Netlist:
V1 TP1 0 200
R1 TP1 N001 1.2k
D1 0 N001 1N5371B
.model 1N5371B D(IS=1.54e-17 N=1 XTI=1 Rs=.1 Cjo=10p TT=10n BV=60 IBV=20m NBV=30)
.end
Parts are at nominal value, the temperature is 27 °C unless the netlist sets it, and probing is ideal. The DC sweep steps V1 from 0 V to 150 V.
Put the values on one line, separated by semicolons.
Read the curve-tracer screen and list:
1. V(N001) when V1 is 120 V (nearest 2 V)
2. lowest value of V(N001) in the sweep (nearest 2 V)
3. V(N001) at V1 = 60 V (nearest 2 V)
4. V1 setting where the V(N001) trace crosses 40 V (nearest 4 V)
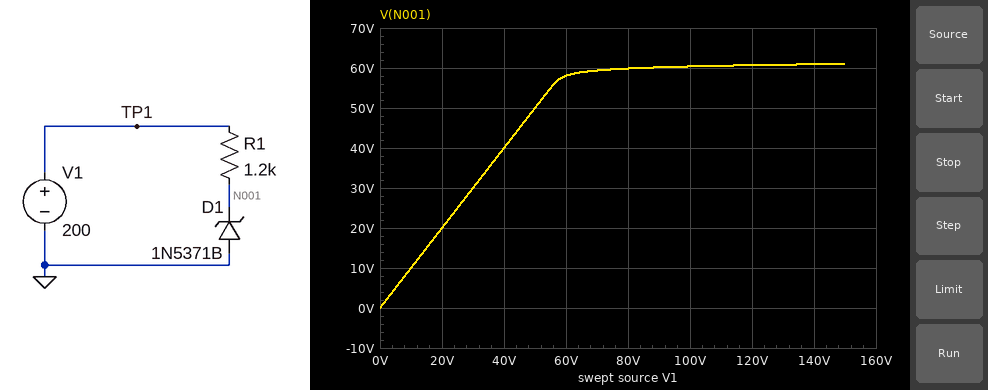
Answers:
60 V; 0 V; 58 V; 40 V
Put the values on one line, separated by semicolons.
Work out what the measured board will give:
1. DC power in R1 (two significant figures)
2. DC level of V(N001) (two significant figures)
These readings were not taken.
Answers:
16 W; 61 V
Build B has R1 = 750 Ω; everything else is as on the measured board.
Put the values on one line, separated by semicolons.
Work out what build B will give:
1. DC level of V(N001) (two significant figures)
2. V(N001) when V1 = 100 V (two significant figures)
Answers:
62 V; 61 V
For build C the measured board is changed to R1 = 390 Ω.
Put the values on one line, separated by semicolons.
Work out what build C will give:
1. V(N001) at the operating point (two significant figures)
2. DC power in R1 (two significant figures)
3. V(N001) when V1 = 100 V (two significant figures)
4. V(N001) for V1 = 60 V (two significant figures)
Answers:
62 V; 49 W; 61 V; 59 V
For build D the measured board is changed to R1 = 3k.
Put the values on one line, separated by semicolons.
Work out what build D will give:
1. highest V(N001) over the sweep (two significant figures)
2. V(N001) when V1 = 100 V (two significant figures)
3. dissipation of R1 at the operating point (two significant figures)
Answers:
60 V; 60 V; 6.5 W
